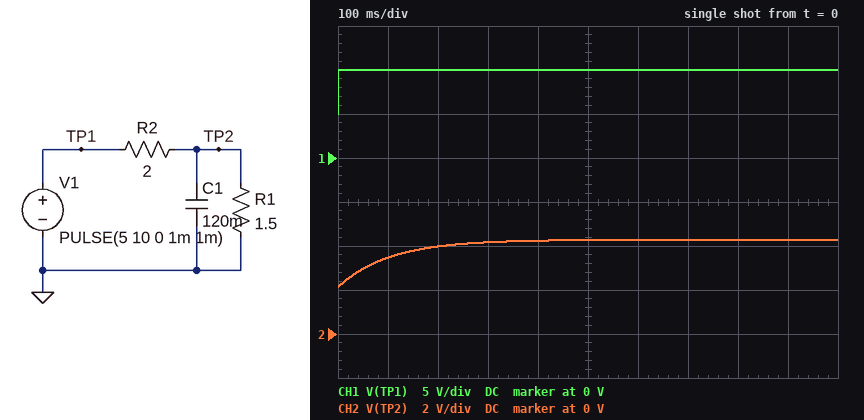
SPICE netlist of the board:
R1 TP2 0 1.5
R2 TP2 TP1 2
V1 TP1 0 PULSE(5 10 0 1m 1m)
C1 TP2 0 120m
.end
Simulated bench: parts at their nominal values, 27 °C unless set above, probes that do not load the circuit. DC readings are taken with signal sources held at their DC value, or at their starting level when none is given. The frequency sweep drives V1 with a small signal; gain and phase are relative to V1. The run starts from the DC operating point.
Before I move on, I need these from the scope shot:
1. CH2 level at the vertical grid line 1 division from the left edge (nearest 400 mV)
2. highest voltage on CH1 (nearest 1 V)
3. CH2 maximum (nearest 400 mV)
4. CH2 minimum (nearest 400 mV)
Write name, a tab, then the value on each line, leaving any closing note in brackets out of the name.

CH2 level at the vertical grid line 1 division from the left edge	3.6 V
highest voltage on CH1	10 V
CH2 maximum	4.4 V
CH2 minimum	2.0 V
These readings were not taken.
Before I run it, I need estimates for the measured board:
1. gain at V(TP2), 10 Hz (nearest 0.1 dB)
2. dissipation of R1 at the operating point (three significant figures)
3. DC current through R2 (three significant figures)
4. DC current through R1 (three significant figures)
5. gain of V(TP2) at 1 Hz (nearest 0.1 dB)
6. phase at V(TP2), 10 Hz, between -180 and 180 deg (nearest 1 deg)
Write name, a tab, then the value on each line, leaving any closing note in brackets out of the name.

gain at V(TP2), 10 Hz	-23.7 dB
dissipation of R1 at the operating point	3.06 W
DC current through R2	1.43 A
DC current through R1	1.43 A
gain of V(TP2) at 1 Hz	-8.9 dB
phase at V(TP2), 10 Hz, between -180 and 180 deg	-81 deg
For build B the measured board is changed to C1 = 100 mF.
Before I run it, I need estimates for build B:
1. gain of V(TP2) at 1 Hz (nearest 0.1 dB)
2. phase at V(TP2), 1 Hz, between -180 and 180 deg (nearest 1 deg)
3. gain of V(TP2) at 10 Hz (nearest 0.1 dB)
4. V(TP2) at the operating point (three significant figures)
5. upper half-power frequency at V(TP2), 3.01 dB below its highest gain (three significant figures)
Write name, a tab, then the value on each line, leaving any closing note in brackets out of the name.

gain of V(TP2) at 1 Hz	-8.5 dB
phase at V(TP2), 1 Hz, between -180 and 180 deg	-28 deg
gain of V(TP2) at 10 Hz	-22.1 dB
V(TP2) at the operating point	2.14 V
upper half-power frequency at V(TP2), 3.01 dB below its highest gain	1.86 Hz
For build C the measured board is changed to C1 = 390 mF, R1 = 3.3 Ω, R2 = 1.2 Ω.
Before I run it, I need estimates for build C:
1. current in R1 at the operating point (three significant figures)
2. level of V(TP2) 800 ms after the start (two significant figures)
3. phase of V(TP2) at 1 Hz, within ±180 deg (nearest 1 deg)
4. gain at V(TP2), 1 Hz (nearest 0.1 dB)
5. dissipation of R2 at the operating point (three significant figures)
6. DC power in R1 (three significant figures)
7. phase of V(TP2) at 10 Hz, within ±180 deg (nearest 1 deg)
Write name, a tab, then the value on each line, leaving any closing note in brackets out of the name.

current in R1 at the operating point	1.11 A
level of V(TP2) 800 ms after the start	7.0 V
phase of V(TP2) at 1 Hz, within ±180 deg	-65 deg
gain at V(TP2), 1 Hz	-10.2 dB
dissipation of R2 at the operating point	1.48 W
DC power in R1	4.07 W
phase of V(TP2) at 10 Hz, within ±180 deg	-87 deg
